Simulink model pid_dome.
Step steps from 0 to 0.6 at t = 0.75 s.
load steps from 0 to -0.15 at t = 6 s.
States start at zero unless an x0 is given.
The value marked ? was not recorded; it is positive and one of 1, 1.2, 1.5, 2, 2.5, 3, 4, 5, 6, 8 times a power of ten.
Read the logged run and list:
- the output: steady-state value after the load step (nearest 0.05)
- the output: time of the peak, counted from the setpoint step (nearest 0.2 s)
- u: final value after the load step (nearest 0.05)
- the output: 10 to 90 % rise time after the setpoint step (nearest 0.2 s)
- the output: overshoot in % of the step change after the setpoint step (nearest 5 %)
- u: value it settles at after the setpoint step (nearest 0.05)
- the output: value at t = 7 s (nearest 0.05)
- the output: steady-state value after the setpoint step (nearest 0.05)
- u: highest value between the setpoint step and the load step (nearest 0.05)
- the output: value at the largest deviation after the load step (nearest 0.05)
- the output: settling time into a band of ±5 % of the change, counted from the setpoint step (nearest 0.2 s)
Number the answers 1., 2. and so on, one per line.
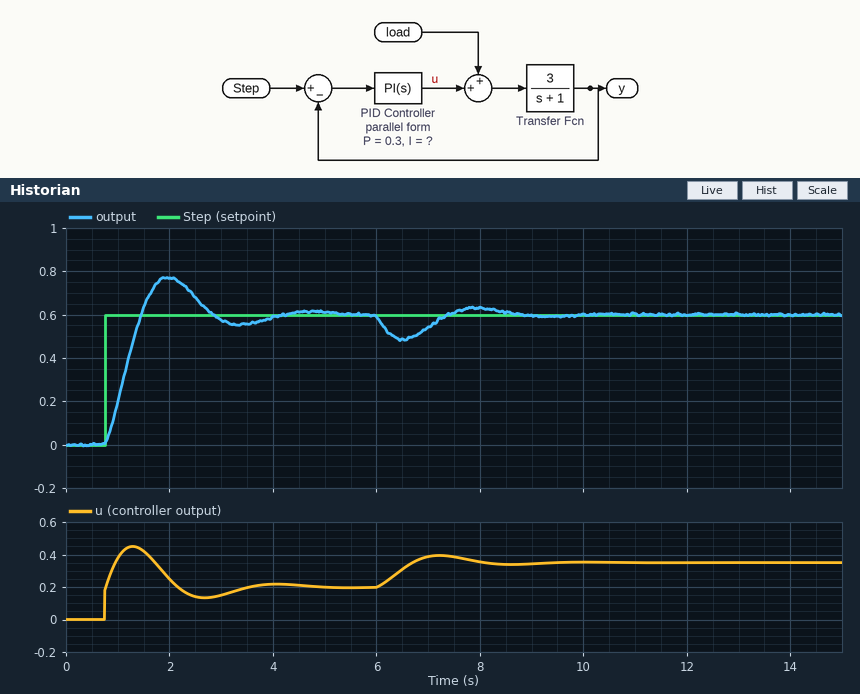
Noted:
1. 0.60
2. 1.2 s
3. 0.35
4. 0.6 s
5. 30 %
6. 0.20
7. 0.55
8. 0.60
9. 0.45
10. 0.50
11. 3.0 s
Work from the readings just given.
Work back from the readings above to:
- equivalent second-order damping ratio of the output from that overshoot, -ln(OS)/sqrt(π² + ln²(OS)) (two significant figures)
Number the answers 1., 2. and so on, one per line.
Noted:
1. 0.36
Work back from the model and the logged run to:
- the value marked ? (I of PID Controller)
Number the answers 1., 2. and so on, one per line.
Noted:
1. 2
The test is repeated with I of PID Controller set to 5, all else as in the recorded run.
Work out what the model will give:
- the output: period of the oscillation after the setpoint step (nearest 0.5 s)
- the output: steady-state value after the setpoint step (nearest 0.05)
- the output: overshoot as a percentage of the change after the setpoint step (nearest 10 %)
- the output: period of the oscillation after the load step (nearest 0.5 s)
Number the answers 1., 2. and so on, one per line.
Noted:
1. 1.5 s
2. 0.60
3. 50 %
4. 1.5 s
